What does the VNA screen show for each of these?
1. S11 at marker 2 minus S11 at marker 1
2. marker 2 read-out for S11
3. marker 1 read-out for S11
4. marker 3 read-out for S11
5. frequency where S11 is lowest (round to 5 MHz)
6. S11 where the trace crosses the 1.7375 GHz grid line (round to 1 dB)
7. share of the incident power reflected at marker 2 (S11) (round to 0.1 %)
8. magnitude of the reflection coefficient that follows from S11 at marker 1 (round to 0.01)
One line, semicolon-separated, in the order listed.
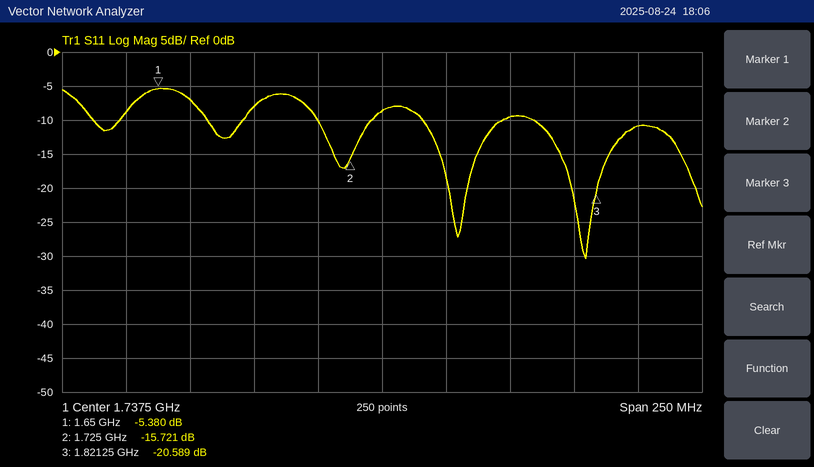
-10.341 dB; -15.721 dB; -5.380 dB; -20.589 dB; 1.815 GHz; -9 dB; 2.7 %; 0.54
